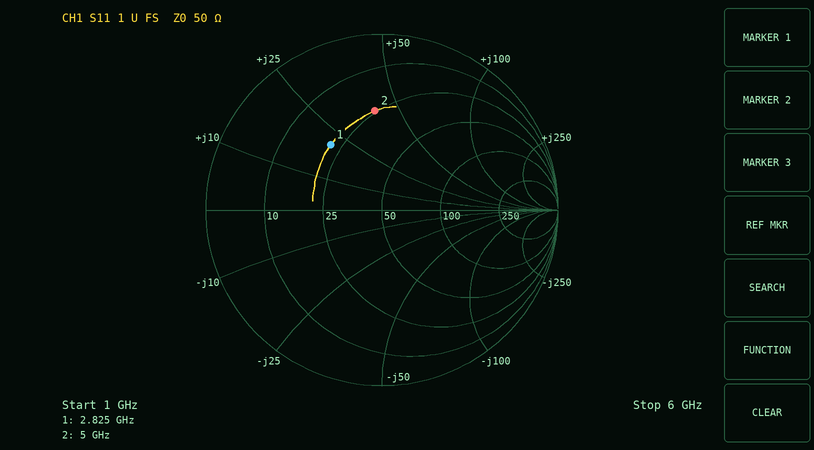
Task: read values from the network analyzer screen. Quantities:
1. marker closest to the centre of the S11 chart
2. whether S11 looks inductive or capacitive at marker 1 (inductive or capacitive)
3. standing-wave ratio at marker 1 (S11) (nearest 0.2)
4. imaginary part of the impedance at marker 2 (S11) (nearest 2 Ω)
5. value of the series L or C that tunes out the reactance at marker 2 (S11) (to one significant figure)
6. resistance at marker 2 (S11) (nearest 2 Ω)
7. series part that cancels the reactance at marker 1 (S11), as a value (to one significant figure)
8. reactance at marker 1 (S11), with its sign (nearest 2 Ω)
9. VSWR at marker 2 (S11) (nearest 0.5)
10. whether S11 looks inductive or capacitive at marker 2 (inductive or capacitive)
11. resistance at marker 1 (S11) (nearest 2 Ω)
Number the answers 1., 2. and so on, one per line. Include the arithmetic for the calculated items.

1. marker 1
2. inductive
3. 2.8
4. +40 Ω
5. C = 1/(2π × 5 GHz × 40 Ω) ≈ 796 fF, so 800 fF to one significant figure
6. 24 Ω
7. C = 1/(2π × 2.825 GHz × 20 Ω) ≈ 3 pF
8. +20 Ω
9. 3.5
10. inductive
11. 22 Ω
